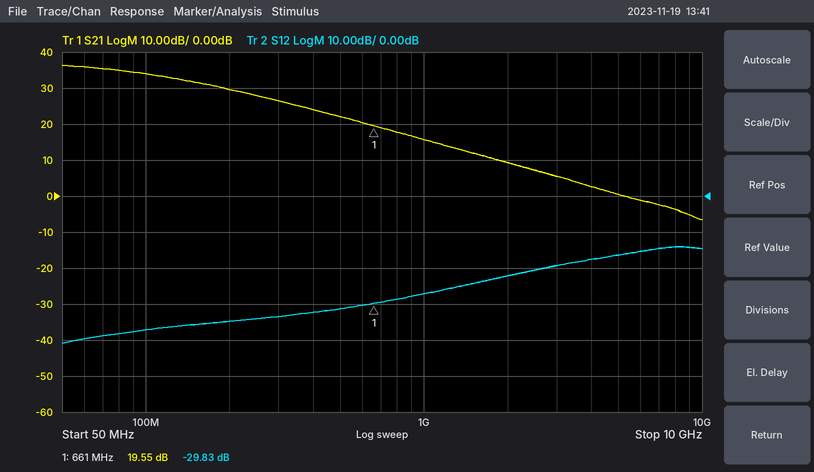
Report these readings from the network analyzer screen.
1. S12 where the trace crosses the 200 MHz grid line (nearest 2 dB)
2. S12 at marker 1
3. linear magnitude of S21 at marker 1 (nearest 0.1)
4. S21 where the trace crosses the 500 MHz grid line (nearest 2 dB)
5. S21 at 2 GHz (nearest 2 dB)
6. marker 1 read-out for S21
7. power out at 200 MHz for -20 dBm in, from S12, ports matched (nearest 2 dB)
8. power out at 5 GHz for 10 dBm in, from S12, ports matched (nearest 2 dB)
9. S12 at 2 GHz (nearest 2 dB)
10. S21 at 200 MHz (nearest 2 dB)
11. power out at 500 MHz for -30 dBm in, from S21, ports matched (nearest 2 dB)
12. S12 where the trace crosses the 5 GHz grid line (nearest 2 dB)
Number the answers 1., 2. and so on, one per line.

1. -34 dB
2. -29.83 dB
3. 9.5
4. 22 dB
5. 10 dB
6. 19.55 dB
7. -54 dBm
8. -6 dBm
9. -22 dB
10. 30 dB
11. -8 dBm
12. -16 dB
